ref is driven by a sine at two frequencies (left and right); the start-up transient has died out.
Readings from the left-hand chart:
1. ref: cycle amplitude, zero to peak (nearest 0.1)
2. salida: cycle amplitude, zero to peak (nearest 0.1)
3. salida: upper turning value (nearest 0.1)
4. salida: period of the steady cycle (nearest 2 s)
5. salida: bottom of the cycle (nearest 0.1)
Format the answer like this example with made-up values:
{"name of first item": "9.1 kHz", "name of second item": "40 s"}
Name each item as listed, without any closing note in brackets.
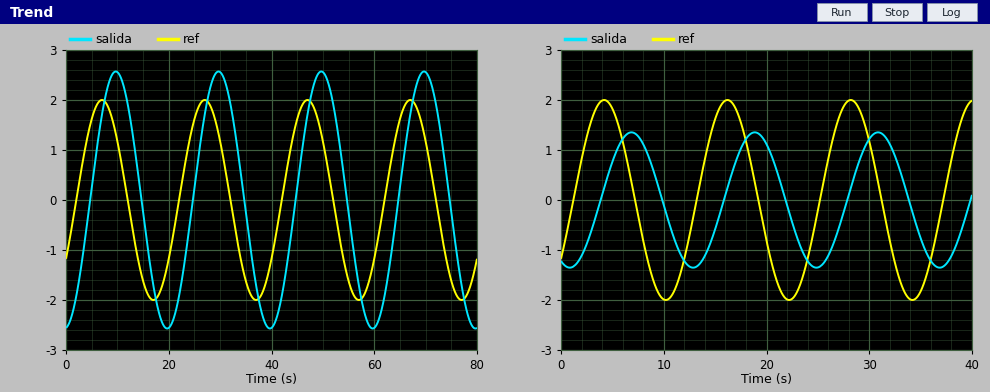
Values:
{"ref: cycle amplitude, zero to peak": "2.0", "salida: cycle amplitude, zero to peak": "2.6", "salida: upper turning value": "2.6", "salida: period of the steady cycle": "20 s", "salida: bottom of the cycle": "-2.6"}
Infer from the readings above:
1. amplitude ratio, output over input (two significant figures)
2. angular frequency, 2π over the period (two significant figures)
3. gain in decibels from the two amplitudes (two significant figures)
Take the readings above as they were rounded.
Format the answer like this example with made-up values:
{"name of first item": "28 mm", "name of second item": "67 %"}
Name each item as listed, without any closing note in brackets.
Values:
{"amplitude ratio, output over input": "1.3", "angular frequency, 2π over the period": "0.31 rad/s", "gain in decibels from the two amplitudes": "2.3 dB"}
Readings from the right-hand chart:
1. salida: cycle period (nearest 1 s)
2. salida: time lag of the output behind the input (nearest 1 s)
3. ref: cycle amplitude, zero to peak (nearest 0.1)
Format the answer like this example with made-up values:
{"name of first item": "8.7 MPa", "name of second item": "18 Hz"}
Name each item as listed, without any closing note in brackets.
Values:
{"salida: cycle period": "12 s", "salida: time lag of the output behind the input": "3 s", "ref: cycle amplitude, zero to peak": "2.0"}
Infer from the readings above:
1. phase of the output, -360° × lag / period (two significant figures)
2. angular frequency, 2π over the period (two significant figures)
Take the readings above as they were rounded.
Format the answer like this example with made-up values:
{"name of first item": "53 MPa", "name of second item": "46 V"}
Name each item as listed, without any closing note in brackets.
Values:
{"phase of the output, -360° × lag / period": "-90°", "angular frequency, 2π over the period": "0.52 rad/s"}
